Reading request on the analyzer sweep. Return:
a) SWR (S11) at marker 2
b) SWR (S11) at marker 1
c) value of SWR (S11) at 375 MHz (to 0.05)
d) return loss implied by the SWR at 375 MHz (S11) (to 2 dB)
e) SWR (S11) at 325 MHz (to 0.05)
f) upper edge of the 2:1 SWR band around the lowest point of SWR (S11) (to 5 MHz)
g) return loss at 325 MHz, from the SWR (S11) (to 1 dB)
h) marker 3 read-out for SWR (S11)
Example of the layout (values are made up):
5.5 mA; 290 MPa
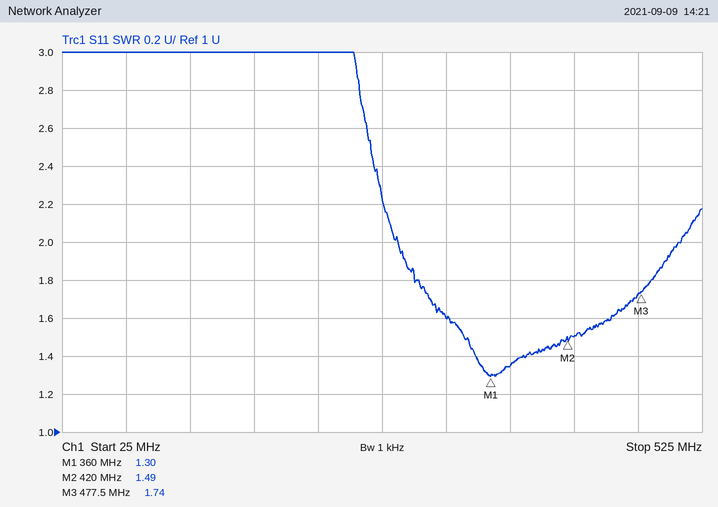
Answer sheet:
1.49; 1.30; 1.35; 16 dB; 1.60; 510 MHz; 13 dB; 1.74
